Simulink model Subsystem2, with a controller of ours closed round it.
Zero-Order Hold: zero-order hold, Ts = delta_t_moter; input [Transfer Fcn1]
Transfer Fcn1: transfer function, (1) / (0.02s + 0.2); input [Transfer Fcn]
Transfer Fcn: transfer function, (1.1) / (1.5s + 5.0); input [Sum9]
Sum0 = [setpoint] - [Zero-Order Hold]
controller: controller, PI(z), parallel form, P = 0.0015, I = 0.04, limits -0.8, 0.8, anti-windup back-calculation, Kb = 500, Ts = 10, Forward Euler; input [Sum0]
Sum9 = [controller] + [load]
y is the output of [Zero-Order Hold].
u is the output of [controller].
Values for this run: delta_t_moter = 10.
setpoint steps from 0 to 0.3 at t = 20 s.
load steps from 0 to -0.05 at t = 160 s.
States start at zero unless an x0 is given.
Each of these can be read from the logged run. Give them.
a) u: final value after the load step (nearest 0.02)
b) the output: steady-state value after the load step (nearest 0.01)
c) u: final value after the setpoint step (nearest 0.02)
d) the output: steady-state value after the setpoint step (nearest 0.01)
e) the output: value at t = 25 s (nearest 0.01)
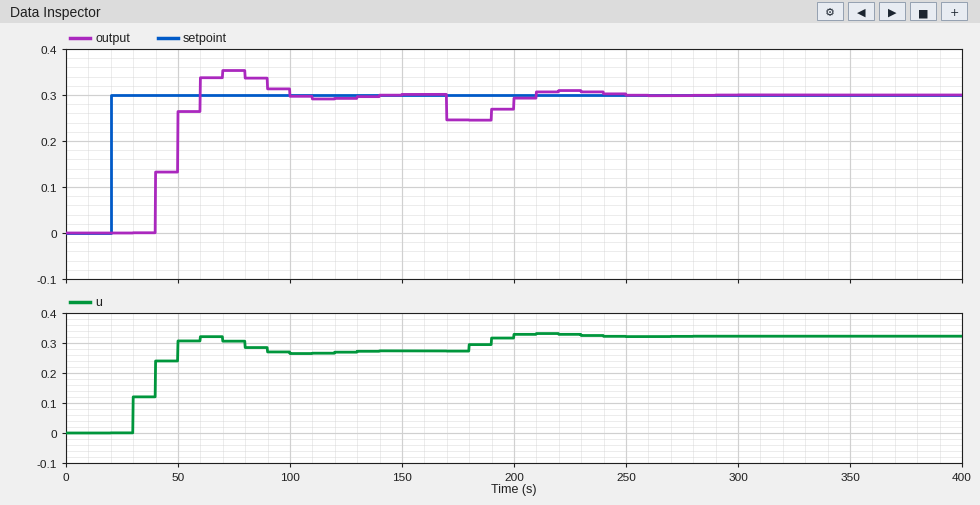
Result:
0.32
0.30
0.28
0.30
0.00
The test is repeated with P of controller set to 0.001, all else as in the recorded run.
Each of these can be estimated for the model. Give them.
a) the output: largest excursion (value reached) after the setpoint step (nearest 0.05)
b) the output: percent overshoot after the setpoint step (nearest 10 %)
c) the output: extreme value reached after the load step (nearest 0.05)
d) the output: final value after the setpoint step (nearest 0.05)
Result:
0.35
20 %
0.25
0.30
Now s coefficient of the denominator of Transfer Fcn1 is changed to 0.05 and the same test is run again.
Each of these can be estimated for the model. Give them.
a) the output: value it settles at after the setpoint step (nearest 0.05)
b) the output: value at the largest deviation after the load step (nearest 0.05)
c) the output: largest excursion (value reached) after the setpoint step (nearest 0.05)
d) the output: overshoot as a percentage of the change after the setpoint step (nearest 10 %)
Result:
0.30
0.25
0.35
20 %
